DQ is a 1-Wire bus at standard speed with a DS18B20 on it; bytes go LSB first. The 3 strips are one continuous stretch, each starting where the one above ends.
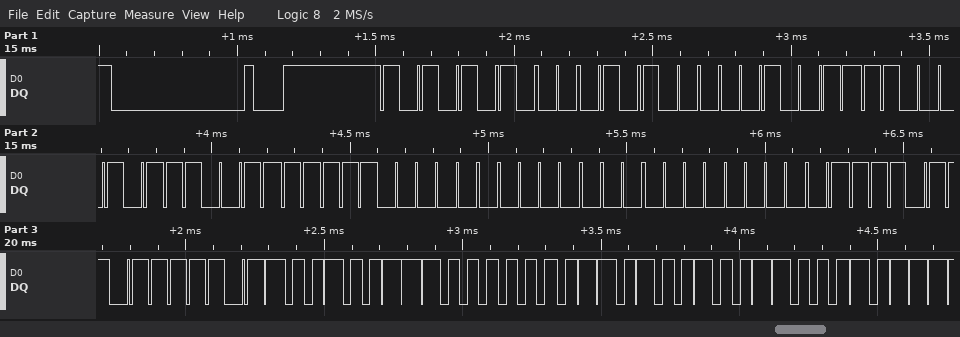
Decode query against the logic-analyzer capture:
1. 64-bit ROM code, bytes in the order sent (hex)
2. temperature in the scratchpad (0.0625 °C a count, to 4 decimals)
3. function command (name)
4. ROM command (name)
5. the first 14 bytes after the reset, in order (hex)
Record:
28 C8 A3 F3 07 00 00 DE
28.5625 °C
Read Scratchpad
Match ROM
55 28 C8 A3 F3 07 00 00 DE BE C9 01 4B 46
